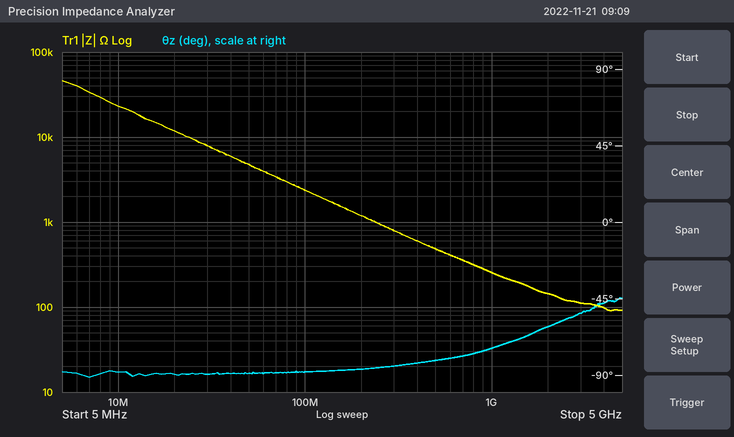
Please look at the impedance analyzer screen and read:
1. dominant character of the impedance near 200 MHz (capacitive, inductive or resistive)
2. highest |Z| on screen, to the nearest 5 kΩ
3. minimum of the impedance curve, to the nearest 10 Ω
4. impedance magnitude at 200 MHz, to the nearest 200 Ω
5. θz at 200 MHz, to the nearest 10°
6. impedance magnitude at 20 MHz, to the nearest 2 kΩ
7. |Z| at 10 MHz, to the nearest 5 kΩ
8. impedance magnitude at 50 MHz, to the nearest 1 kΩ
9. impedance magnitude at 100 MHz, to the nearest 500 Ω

capacitive
45 kΩ
90 Ω
1.2 kΩ
-90°
12 kΩ
25 kΩ
5 kΩ
2.5 kΩ
